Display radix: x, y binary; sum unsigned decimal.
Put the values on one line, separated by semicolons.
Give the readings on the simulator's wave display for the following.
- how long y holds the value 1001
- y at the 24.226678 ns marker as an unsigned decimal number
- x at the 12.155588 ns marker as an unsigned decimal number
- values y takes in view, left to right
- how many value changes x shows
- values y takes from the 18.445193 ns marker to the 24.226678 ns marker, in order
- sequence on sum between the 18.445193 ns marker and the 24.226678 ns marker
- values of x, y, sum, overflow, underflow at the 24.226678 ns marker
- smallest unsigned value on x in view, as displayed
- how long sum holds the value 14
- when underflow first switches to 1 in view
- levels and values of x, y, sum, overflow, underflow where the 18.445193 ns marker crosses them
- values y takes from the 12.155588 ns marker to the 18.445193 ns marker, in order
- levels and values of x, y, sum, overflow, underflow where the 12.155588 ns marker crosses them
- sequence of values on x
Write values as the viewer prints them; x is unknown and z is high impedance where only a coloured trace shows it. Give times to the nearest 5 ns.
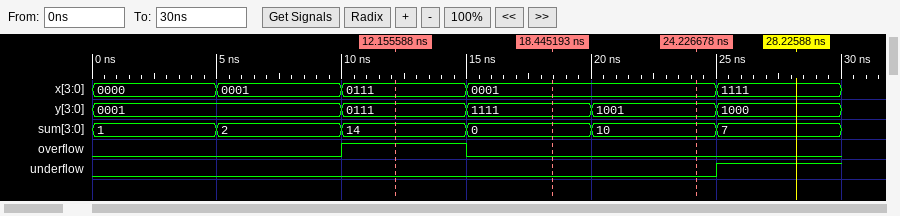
5 ns; 9; 7; 0001, 0111, 1111, 1001, 1000; 4; 1111, 1001; 0, 10; x=0001, y=1001, sum=10, overflow=0, underflow=0; 0000; 5 ns; 25 ns; x=0001, y=1111, sum=0, overflow=0, underflow=0; 0111, 1111; x=0111, y=0111, sum=14, overflow=1, underflow=0; 0000, 0001, 0111, 0001, 1111
